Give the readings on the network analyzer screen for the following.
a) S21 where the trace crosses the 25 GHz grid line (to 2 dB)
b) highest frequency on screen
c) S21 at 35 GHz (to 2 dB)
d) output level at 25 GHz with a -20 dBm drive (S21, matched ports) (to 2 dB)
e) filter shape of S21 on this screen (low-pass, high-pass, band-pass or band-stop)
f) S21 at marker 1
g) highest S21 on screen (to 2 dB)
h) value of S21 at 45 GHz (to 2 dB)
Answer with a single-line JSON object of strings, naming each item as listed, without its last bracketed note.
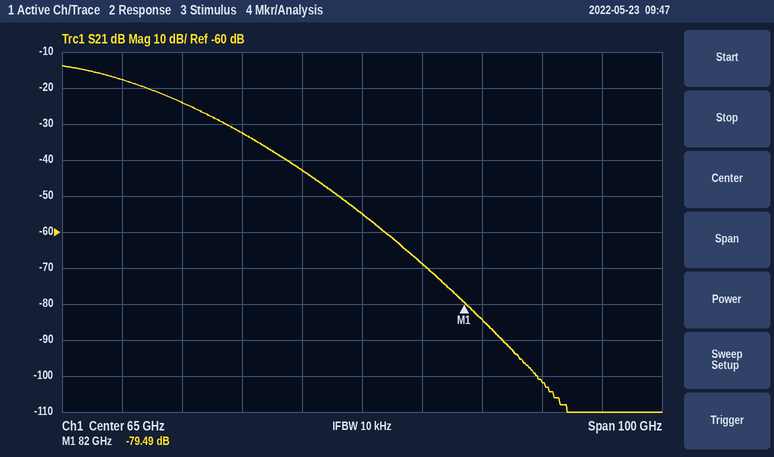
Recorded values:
{"S21 where the trace crosses the 25 GHz grid line": "-18 dB", "highest frequency on screen": "115 GHz", "S21 at 35 GHz": "-24 dB", "output level at 25 GHz with a -20 dBm drive (S21, matched ports)": "-38 dBm", "filter shape of S21 on this screen": "low-pass", "S21 at marker 1": "-79.49 dB", "highest S21 on screen": "-14 dB", "value of S21 at 45 GHz": "-32 dB"}
